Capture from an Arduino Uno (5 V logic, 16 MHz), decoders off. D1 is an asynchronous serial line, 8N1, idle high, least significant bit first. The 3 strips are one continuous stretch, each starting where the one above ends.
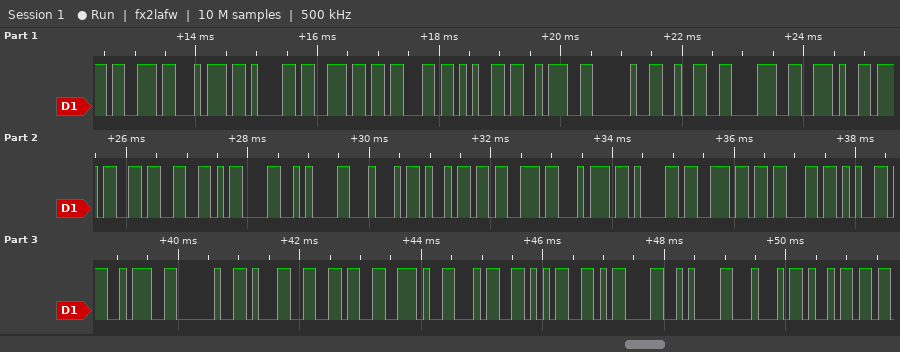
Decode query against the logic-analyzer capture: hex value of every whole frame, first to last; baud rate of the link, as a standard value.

73 74 61 6E 63 65 3A 20 32 38 2E 37 33 0D 0A 44 69 73 74 61 6E 63 65 3A 20 31 36 2E 34 35 0D 0A 44 69
9600 baud
